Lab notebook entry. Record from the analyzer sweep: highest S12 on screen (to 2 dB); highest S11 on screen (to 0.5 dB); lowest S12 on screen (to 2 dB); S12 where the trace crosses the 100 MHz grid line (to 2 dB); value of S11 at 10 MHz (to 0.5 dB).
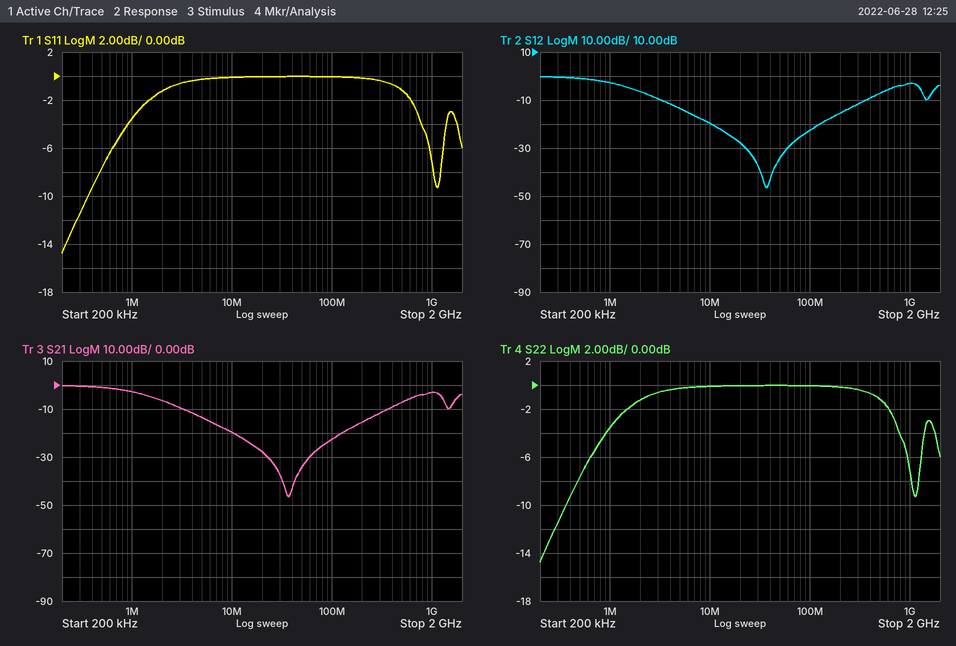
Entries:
0 dB
0.0 dB
-46 dB
-22 dB
0.0 dB
